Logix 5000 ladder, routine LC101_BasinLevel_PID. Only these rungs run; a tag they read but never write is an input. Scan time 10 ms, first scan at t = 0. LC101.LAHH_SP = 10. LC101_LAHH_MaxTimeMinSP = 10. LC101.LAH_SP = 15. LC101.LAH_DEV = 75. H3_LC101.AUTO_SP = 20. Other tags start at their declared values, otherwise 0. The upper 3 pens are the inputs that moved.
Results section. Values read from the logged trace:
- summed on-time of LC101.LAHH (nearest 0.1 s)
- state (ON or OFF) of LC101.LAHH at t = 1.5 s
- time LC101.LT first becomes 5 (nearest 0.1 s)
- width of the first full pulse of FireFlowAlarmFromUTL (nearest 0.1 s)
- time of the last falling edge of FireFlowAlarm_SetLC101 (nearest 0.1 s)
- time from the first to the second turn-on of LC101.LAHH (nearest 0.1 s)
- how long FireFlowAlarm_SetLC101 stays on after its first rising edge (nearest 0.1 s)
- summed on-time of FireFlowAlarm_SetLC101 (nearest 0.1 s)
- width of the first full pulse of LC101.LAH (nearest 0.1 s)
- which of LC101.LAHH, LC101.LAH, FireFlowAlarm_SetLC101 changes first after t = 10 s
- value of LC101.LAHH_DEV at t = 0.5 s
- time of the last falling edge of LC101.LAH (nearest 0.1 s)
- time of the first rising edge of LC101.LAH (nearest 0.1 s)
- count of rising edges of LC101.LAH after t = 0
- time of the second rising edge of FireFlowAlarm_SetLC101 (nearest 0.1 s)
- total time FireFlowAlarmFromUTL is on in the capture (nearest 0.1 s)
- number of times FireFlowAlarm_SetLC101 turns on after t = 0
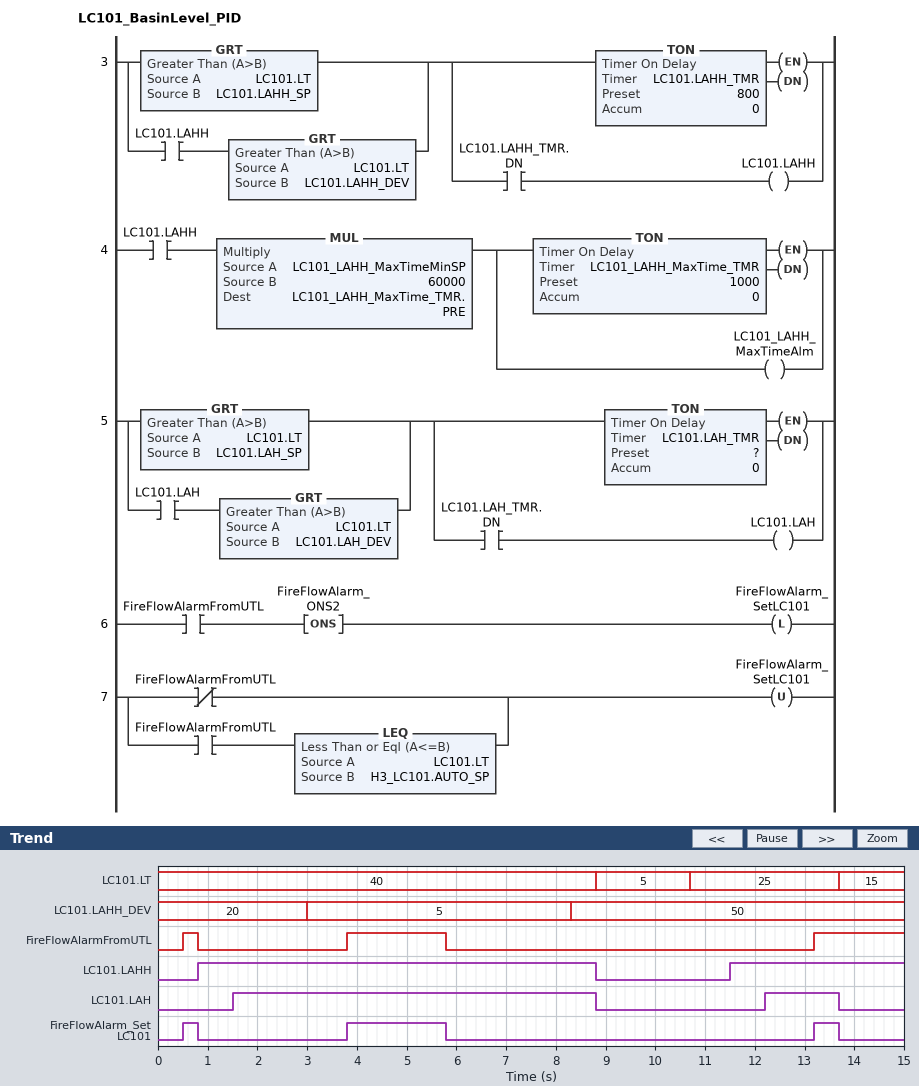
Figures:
11.5 s
ON
8.8 s
0.3 s
13.7 s
10.7 s
0.3 s
2.8 s
7.3 s
LC101.LAHH
20
13.7 s
1.5 s
2
3.8 s
4.1 s
3
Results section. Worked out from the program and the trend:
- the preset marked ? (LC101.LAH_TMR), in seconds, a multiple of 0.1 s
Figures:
1.5 s
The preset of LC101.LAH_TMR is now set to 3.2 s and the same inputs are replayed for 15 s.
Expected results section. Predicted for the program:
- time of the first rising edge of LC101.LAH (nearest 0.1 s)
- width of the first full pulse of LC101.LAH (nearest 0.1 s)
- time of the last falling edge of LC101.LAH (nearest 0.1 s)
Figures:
3.2 s
5.6 s
8.8 s
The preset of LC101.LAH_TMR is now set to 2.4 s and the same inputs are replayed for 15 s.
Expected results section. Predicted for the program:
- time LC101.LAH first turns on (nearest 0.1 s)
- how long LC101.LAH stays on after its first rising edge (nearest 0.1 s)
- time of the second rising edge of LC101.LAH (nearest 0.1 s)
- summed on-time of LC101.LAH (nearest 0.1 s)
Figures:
2.4 s
6.4 s
13.1 s
7.0 s
